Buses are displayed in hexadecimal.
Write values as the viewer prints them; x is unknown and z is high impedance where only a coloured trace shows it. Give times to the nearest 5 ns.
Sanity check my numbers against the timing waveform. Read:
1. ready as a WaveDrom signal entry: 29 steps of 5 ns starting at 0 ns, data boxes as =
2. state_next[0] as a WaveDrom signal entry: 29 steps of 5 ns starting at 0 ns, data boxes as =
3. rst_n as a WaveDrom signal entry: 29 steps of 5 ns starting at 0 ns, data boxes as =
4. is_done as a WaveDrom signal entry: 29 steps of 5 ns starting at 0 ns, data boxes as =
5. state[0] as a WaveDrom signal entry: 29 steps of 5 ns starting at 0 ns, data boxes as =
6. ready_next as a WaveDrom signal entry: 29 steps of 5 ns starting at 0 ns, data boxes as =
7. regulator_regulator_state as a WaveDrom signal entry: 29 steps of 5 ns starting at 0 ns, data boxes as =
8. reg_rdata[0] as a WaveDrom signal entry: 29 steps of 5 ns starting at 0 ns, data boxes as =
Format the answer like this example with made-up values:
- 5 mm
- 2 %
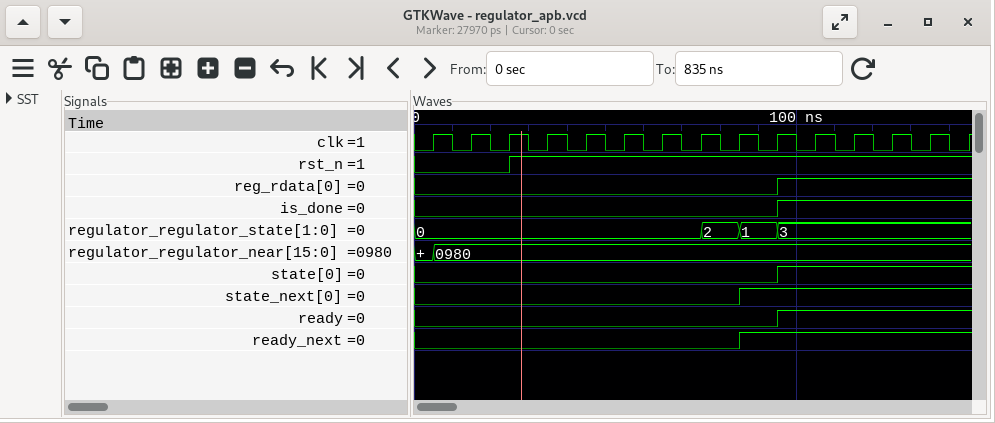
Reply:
- {name: 'ready', wave: '0..................1.........'}
- {name: 'state_next[0]', wave: '0................1...........'}
- {name: 'rst_n', wave: '0....1.......................'}
- {name: 'is_done', wave: '0..................1.........'}
- {name: 'state[0]', wave: '0..................1.........'}
- {name: 'ready_next', wave: '0................1...........'}
- {name: 'regulator_regulator_state', wave: '=..............=.=.=.........', data: '0 2 1 3'}
- {name: 'reg_rdata[0]', wave: '0..................1.........'}
